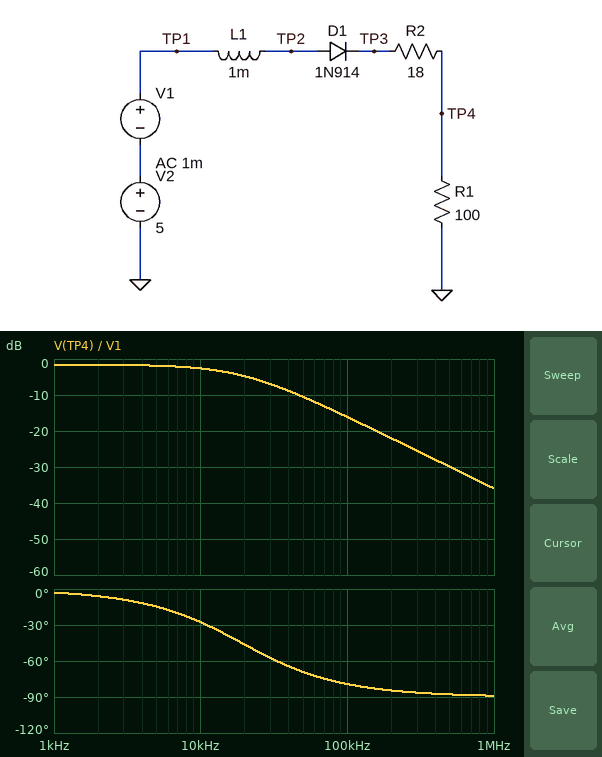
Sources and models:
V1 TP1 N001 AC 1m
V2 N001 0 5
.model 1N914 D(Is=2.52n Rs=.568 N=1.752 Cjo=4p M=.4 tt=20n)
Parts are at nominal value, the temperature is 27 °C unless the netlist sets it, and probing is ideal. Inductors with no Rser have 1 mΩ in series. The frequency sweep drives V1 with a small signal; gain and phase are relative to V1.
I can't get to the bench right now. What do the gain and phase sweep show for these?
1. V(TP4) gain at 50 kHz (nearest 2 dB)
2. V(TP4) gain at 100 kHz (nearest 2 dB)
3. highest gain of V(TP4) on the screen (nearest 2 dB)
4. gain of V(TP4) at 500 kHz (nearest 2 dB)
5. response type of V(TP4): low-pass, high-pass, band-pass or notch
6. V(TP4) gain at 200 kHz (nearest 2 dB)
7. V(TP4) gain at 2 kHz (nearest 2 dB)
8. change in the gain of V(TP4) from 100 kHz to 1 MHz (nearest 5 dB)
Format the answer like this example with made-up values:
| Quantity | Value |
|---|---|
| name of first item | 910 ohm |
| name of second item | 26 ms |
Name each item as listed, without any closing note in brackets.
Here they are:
| Quantity | Value |
|---|---|
| V(TP4) gain at 50 kHz | -10 dB |
| V(TP4) gain at 100 kHz | -16 dB |
| highest gain of V(TP4) on the screen | -2 dB |
| gain of V(TP4) at 500 kHz | -30 dB |
| response type of V(TP4): low-pass, high-pass, band-pass or notch | low-pass |
| V(TP4) gain at 200 kHz | -22 dB |
| V(TP4) gain at 2 kHz | -2 dB |
| change in the gain of V(TP4) from 100 kHz to 1 MHz | -20 dB |
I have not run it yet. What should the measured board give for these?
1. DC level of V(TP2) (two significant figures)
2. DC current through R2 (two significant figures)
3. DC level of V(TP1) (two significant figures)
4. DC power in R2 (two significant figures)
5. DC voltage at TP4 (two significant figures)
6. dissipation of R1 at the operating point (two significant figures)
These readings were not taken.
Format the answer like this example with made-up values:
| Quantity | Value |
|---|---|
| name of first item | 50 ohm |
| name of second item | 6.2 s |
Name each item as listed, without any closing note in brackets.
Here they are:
| Quantity | Value |
|---|---|
| DC level of V(TP2) | 5.0 V |
| DC current through R2 | 36 mA |
| DC level of V(TP1) | 5.0 V |
| DC power in R2 | 23 mW |
| DC voltage at TP4 | 3.6 V |
| dissipation of R1 at the operating point | 130 mW |
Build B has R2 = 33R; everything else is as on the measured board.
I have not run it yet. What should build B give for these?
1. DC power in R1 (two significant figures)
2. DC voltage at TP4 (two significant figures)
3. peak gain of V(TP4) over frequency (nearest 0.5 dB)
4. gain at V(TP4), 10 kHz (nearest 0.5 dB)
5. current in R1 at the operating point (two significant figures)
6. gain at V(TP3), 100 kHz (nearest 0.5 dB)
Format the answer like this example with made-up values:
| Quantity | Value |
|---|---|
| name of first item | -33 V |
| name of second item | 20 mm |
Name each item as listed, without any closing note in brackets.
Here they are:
| Quantity | Value |
|---|---|
| DC power in R1 | 100 mW |
| DC voltage at TP4 | 3.2 V |
| peak gain of V(TP4) over frequency | -2.5 dB |
| gain at V(TP4), 10 kHz | -3.5 dB |
| current in R1 at the operating point | 32 mA |
| gain at V(TP3), 100 kHz | -13.5 dB |
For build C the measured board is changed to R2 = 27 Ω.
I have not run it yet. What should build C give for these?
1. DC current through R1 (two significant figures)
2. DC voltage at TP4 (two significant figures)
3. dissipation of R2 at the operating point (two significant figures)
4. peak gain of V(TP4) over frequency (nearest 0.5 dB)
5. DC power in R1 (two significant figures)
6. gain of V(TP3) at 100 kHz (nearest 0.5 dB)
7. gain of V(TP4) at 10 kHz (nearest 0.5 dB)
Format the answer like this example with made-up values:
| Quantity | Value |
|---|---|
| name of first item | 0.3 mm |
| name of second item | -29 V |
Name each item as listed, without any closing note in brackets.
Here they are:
| Quantity | Value |
|---|---|
| DC current through R1 | 33 mA |
| DC voltage at TP4 | 3.3 V |
| dissipation of R2 at the operating point | 30 mW |
| peak gain of V(TP4) over frequency | -2.0 dB |
| DC power in R1 | 110 mW |
| gain of V(TP3) at 100 kHz | -14.0 dB |
| gain of V(TP4) at 10 kHz | -3.0 dB |
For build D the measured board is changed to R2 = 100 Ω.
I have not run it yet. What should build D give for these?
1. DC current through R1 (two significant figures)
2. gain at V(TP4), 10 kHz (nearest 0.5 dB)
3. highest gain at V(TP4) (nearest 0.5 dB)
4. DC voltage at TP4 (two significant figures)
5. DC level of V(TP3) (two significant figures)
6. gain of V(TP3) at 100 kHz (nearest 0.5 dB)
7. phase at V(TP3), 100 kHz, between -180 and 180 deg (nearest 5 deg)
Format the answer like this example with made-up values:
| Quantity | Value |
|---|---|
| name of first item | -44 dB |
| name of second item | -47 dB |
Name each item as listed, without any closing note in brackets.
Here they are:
| Quantity | Value |
|---|---|
| DC current through R1 | 21 mA |
| gain at V(TP4), 10 kHz | -6.5 dB |
| highest gain at V(TP4) | -6.0 dB |
| DC voltage at TP4 | 2.1 V |
| DC level of V(TP3) | 4.3 V |
| gain of V(TP3) at 100 kHz | -10.5 dB |
| phase at V(TP3), 100 kHz, between -180 and 180 deg | -70 deg |
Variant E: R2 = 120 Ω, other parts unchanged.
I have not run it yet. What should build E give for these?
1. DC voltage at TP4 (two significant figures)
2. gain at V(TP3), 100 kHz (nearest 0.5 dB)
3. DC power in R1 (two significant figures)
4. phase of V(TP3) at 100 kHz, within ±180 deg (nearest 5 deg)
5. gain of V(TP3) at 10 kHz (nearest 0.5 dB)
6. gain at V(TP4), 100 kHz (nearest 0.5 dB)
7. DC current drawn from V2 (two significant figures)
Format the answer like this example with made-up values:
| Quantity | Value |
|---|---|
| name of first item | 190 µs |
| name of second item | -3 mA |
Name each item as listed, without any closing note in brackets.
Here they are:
| Quantity | Value |
|---|---|
| DC voltage at TP4 | 1.9 V |
| gain at V(TP3), 100 kHz | -9.5 dB |
| DC power in R1 | 38 mW |
| phase of V(TP3) at 100 kHz, within ±180 deg | -70 deg |
| gain of V(TP3) at 10 kHz | -0.5 dB |
| gain at V(TP4), 100 kHz | -16.5 dB |
| DC current drawn from V2 | 19 mA |
